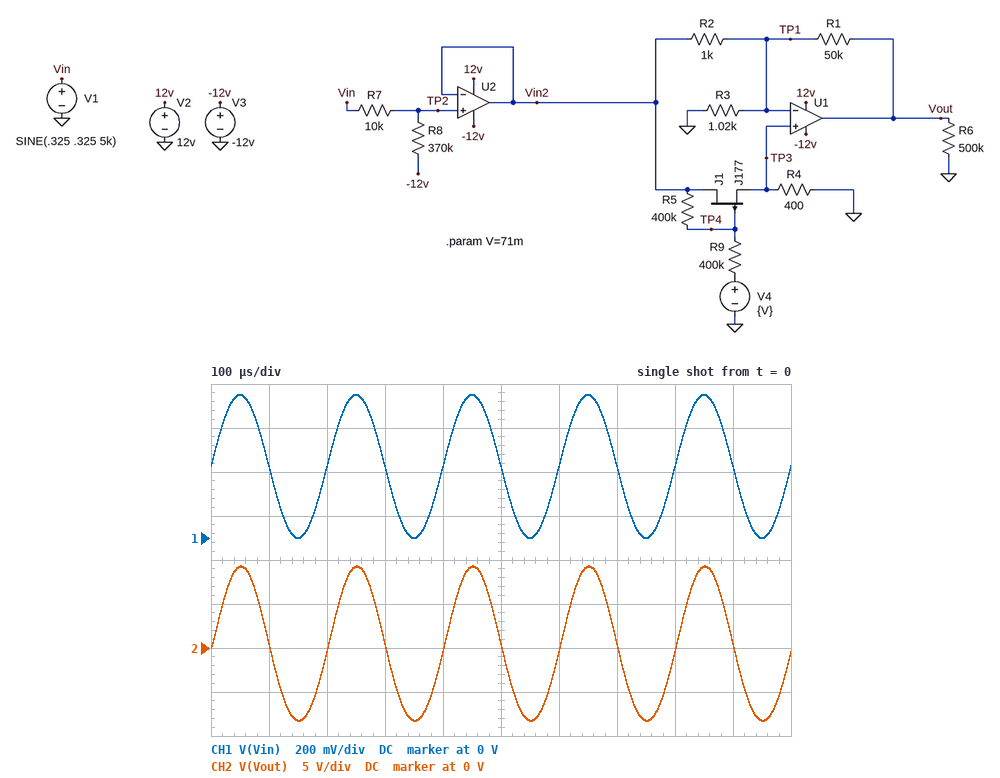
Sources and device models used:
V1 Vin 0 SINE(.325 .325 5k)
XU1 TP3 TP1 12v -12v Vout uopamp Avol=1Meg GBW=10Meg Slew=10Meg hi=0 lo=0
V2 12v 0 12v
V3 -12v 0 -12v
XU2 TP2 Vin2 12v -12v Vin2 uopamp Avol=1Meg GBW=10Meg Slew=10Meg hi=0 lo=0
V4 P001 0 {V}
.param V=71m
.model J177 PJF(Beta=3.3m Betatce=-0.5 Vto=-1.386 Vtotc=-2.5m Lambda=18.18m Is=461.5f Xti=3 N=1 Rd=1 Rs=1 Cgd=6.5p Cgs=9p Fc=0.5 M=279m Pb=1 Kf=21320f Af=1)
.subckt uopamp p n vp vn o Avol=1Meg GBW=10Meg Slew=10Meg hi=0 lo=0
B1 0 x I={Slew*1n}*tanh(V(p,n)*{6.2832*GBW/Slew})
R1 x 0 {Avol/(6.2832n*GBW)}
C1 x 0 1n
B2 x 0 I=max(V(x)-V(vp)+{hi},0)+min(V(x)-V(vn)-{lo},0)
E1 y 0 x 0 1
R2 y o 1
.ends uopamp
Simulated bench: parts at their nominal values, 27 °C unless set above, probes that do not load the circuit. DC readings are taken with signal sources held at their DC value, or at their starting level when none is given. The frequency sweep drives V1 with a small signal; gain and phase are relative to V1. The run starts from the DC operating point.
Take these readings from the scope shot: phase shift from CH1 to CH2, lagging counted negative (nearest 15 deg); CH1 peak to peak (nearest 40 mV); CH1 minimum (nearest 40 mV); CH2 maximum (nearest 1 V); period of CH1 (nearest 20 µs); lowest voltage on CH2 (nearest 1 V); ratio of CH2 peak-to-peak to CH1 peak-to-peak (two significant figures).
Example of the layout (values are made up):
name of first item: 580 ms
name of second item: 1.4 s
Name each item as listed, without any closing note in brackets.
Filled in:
phase shift from CH1 to CH2, lagging counted negative: 0 deg
CH1 peak to peak: 640 mV
CH1 minimum: 0 V
CH2 maximum: 9 V
period of CH1: 200 µs
lowest voltage on CH2: -8 V
ratio of CH2 peak-to-peak to CH1 peak-to-peak: 27
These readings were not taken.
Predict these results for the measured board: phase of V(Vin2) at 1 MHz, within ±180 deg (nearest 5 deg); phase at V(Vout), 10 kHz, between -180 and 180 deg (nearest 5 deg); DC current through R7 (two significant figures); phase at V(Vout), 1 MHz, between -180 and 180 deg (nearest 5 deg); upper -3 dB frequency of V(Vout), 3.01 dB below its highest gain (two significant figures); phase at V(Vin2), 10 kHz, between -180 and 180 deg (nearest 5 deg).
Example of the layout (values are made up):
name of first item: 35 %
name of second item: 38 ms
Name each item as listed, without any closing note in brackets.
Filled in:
phase of V(Vin2) at 1 MHz, within ±180 deg: -5 deg
phase at V(Vout), 10 kHz, between -180 and 180 deg: -5 deg
DC current through R7: 32 µA
phase at V(Vout), 1 MHz, between -180 and 180 deg: -90 deg
upper -3 dB frequency of V(Vout), 3.01 dB below its highest gain: 100 kHz
phase at V(Vin2), 10 kHz, between -180 and 180 deg: 0 deg
